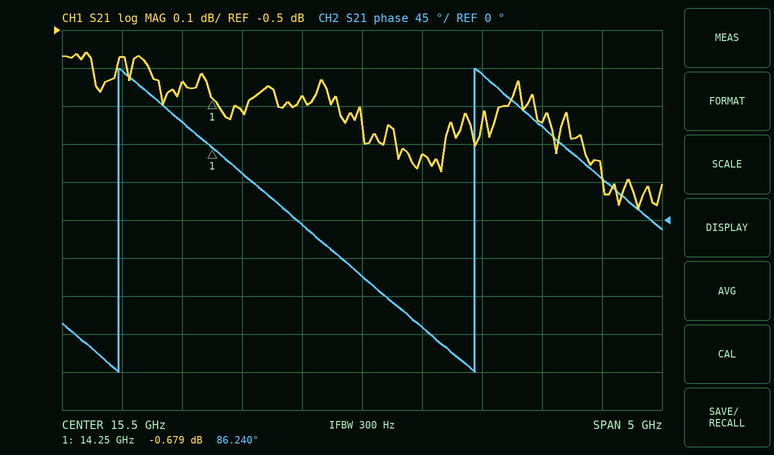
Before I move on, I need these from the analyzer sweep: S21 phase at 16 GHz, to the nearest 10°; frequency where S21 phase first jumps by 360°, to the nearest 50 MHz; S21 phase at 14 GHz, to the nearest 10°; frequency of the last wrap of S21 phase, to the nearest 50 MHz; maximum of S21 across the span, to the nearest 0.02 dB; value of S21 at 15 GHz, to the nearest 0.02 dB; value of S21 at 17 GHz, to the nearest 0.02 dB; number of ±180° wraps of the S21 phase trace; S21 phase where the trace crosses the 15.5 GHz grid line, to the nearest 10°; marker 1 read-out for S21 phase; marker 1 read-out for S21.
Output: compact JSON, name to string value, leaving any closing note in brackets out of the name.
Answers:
{"S21 phase at 16 GHz, to the nearest 10°": "-130°", "frequency where S21 phase first jumps by 360°, to the nearest 50 MHz": "13.45 GHz", "S21 phase at 14 GHz, to the nearest 10°": "120°", "frequency of the last wrap of S21 phase, to the nearest 50 MHz": "16.45 GHz", "maximum of S21 across the span, to the nearest 0.02 dB": "-0.56 dB", "value of S21 at 15 GHz, to the nearest 0.02 dB": "-0.68 dB", "value of S21 at 17 GHz, to the nearest 0.02 dB": "-0.74 dB", "number of ±180° wraps of the S21 phase trace": "2", "S21 phase where the trace crosses the 15.5 GHz grid line, to the nearest 10°": "-70°", "marker 1 read-out for S21 phase": "86.240°", "marker 1 read-out for S21": "-0.679 dB"}
